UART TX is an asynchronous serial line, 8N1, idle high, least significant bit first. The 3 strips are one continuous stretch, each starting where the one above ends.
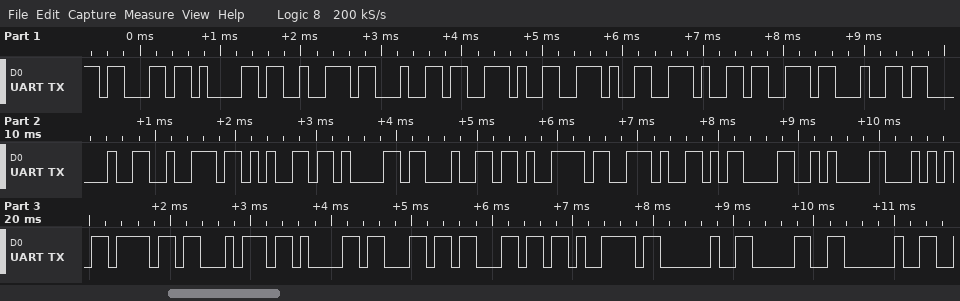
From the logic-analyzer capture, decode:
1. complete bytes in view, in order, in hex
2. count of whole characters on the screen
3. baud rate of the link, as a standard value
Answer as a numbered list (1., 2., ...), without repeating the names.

1. 63 61 72 64 2E 2E 2E 73 64 20 72 65 61 64 79 2E 0D 0A 54 6F 74 61 6C 6C 79 20 30 20
2. 28
3. 9600 baud
